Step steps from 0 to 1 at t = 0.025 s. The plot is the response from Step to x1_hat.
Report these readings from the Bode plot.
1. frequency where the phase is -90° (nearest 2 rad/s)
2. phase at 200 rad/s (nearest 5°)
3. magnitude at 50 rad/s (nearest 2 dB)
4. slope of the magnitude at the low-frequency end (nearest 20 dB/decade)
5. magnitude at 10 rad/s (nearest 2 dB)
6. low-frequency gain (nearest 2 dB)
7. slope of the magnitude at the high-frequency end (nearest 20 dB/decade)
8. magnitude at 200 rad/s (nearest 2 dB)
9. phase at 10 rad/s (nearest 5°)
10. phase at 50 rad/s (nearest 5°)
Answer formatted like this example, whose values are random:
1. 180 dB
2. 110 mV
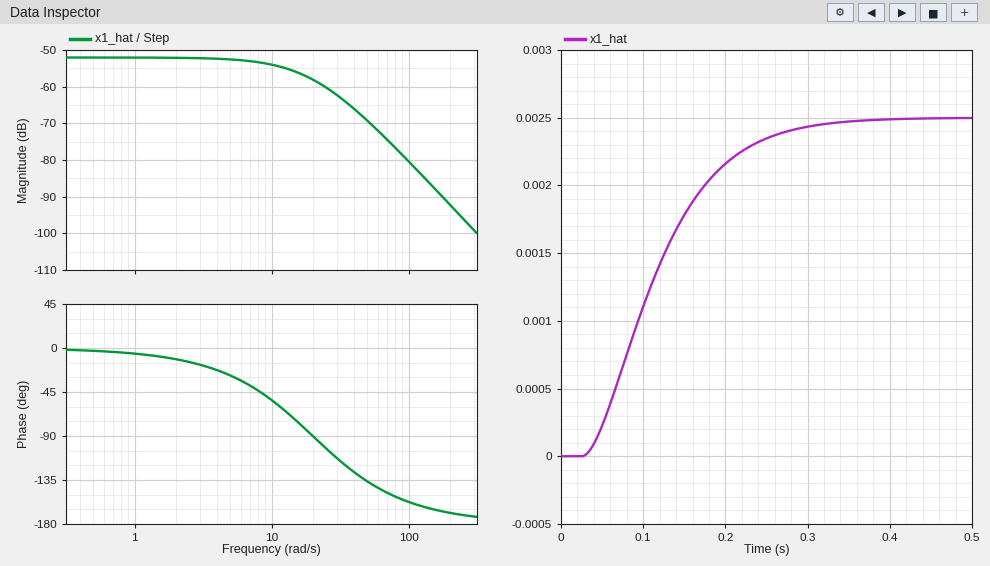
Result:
1. 20 rad/s
2. -170°
3. -70 dB
4. 0 dB/decade
5. -54 dB
6. -52 dB
7. -40 dB/decade
8. -92 dB
9. -55°
10. -135°
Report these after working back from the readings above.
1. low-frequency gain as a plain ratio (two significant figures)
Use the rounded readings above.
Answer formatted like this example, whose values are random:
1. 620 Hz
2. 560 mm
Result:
1. 0.0025
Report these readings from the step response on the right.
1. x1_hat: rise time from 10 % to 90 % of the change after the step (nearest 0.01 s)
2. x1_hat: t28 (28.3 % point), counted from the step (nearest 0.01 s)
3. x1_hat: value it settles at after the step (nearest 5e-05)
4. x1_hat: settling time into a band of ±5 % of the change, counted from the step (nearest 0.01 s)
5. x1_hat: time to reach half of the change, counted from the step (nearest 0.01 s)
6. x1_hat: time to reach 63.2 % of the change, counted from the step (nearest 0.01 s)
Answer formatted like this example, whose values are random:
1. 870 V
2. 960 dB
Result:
1. 0.17 s
2. 0.05 s
3. 0.00250
4. 0.24 s
5. 0.08 s
6. 0.11 s
